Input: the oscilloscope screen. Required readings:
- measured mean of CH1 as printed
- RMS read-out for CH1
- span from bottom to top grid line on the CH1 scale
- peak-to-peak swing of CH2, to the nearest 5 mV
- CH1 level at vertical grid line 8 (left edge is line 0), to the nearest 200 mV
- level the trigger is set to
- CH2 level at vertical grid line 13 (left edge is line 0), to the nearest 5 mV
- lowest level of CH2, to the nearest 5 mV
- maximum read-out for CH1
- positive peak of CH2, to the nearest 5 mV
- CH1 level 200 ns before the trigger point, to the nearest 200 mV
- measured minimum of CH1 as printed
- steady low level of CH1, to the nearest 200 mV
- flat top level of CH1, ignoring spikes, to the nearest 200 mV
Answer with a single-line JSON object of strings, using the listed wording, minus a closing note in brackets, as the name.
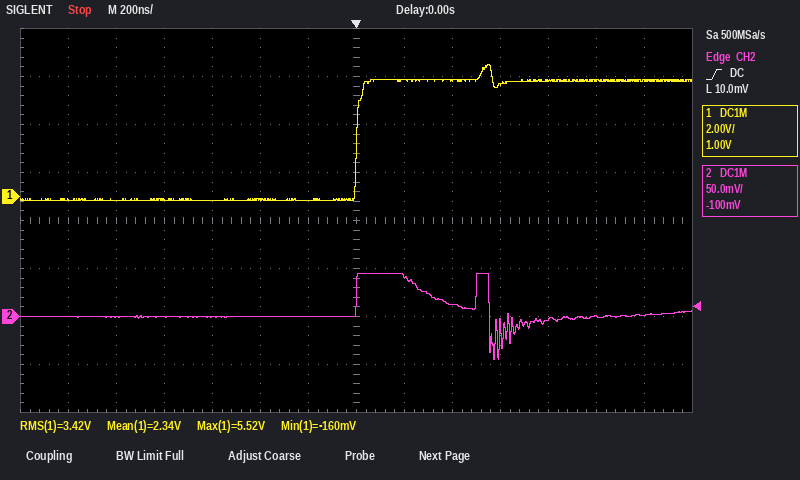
{"measured mean of CH1 as printed": "2.34 V", "RMS read-out for CH1": "3.42 V", "span from bottom to top grid line on the CH1 scale": "16 V", "peak-to-peak swing of CH2, to the nearest 5 mV": "90 mV", "CH1 level at vertical grid line 8 (left edge is line 0), to the nearest 200 mV": "4.8 V", "level the trigger is set to": "10.0 mV", "CH2 level at vertical grid line 13 (left edge is line 0), to the nearest 5 mV": "0 mV", "lowest level of CH2, to the nearest 5 mV": "-45 mV", "maximum read-out for CH1": "5.52 V", "positive peak of CH2, to the nearest 5 mV": "45 mV", "CH1 level 200 ns before the trigger point, to the nearest 200 mV": "-200 mV", "measured minimum of CH1 as printed": "-160 mV", "steady low level of CH1, to the nearest 200 mV": "-200 mV", "flat top level of CH1, ignoring spikes, to the nearest 200 mV": "4.8 V"}
